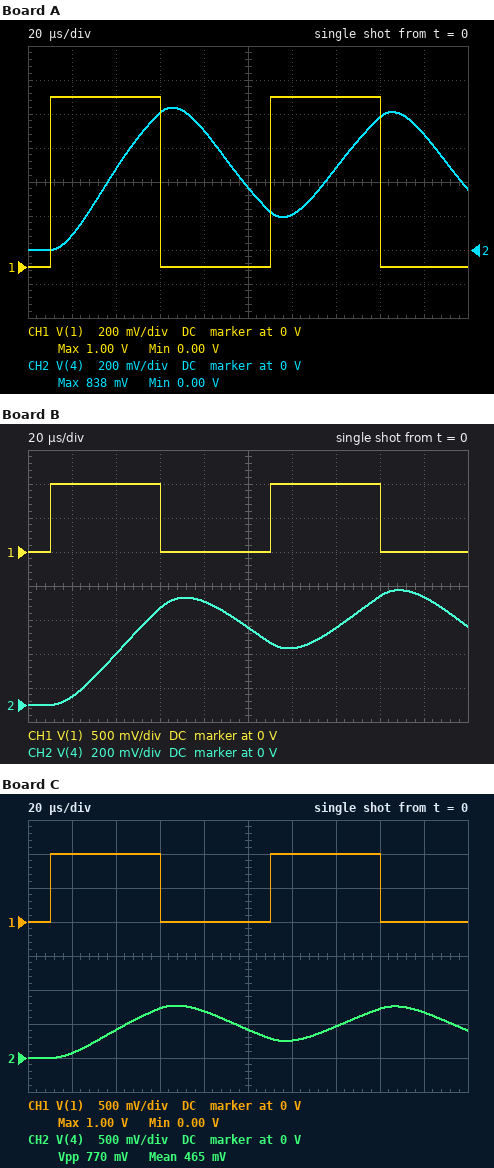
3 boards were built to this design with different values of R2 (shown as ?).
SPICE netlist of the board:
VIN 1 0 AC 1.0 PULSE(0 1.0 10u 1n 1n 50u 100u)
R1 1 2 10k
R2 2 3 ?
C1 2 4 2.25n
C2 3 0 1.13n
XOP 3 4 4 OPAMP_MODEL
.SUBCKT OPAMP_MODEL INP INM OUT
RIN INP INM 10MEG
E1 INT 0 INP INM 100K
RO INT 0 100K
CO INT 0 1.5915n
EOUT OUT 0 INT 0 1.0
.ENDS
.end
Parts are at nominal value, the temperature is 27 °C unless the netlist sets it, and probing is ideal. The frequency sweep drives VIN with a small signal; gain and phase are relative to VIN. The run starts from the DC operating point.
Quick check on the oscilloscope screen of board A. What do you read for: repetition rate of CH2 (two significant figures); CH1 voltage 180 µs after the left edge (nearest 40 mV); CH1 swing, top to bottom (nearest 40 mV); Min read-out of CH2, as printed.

10 kHz
0 V
1.00 V
0.00 V
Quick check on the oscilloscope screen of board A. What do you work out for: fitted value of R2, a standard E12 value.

18 kΩ
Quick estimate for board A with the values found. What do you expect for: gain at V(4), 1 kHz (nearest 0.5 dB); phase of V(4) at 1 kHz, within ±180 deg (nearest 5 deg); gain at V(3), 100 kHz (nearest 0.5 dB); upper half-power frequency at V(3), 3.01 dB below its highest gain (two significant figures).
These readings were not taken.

0 dB
-10 deg
-45.0 dB
7.1 kHz
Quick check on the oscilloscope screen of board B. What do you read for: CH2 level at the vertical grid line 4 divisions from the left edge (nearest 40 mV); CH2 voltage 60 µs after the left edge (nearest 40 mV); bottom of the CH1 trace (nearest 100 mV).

600 mV
560 mV
0 V
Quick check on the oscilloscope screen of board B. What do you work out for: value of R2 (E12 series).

33 kΩ
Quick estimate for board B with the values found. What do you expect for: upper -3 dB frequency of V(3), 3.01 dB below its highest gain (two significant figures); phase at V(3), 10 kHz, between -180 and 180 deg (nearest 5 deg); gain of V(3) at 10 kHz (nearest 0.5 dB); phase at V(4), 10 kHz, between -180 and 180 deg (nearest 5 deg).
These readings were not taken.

4.5 kHz
-125 deg
-11.5 dB
-125 deg
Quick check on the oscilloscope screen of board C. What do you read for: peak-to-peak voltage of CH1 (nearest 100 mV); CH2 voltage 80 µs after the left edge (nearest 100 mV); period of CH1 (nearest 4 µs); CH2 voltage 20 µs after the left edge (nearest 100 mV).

1.0 V
700 mV
100 µs
100 mV
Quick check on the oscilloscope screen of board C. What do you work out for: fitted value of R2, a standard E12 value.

22 kΩ
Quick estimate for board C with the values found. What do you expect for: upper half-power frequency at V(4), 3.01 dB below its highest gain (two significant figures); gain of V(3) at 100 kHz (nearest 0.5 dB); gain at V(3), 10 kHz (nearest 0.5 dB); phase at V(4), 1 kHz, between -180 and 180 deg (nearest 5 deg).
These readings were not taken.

6.2 kHz
-47.0 dB
-8.0 dB
-15 deg
